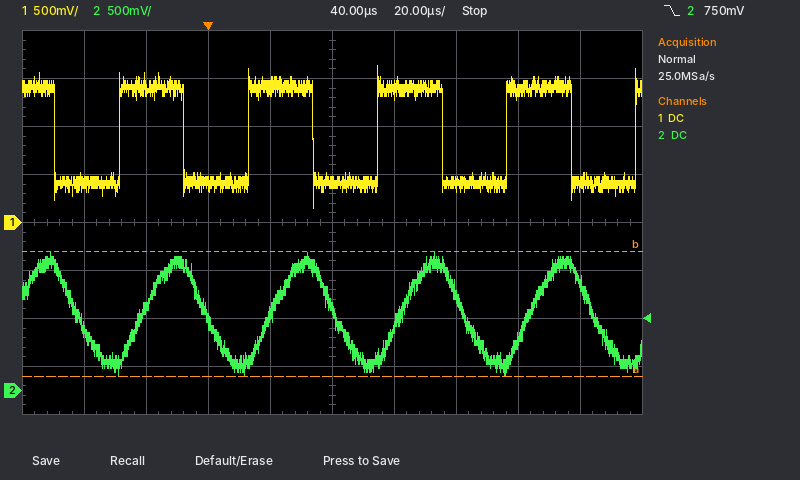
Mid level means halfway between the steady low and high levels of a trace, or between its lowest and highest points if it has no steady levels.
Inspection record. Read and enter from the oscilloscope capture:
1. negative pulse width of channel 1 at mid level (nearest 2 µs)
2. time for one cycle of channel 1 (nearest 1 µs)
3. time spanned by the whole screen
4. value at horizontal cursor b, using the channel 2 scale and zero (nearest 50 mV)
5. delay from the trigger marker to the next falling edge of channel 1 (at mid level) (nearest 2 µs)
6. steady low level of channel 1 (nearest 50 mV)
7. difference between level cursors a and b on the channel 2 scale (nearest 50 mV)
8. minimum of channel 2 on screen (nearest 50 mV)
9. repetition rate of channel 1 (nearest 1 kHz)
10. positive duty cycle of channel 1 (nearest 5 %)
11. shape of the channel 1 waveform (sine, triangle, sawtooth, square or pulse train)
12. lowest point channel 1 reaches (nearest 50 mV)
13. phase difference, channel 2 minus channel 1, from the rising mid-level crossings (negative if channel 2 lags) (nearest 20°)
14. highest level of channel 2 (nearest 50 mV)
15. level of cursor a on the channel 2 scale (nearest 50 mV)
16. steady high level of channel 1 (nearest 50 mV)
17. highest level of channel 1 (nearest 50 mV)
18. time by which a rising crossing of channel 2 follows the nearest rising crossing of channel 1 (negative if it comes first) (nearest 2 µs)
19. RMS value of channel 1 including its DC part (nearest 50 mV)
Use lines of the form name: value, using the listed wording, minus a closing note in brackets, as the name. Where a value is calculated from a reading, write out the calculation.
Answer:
negative pulse width of channel 1 at mid level: 20 µs
time for one cycle of channel 1: 42 µs
time spanned by the whole screen: 200 µs
value at horizontal cursor b, using the channel 2 scale and zero: 1.45 V
delay from the trigger marker to the next falling edge of channel 1 (at mid level): 34 µs
steady low level of channel 1: 400 mV
difference between level cursors a and b on the channel 2 scale: 1.30 V
minimum of channel 2 on screen: 150 mV
repetition rate of channel 1: 1 / 42 µs ≈ 24 kHz
positive duty cycle of channel 1: 50 %
shape of the channel 1 waveform: square
lowest point channel 1 reaches: 150 mV
phase difference, channel 2 minus channel 1, from the rising mid-level crossings (negative if channel 2 lags): −360° × (+8 µs) / 42 µs ≈ -68.6°, so -60° to the nearest 20°
highest level of channel 2: 1.45 V
level of cursor a on the channel 2 scale: 150 mV
steady high level of channel 1: 1.40 V
highest level of channel 1: 1.65 V
time by which a rising crossing of channel 2 follows the nearest rising crossing of channel 1 (negative if it comes first): +8 µs
RMS value of channel 1 including its DC part: √(0.5 × (1.40 V)² + 0.5 × (400 mV)²) ≈ 1.03 V, so 1.05 V to the nearest 50 mV
